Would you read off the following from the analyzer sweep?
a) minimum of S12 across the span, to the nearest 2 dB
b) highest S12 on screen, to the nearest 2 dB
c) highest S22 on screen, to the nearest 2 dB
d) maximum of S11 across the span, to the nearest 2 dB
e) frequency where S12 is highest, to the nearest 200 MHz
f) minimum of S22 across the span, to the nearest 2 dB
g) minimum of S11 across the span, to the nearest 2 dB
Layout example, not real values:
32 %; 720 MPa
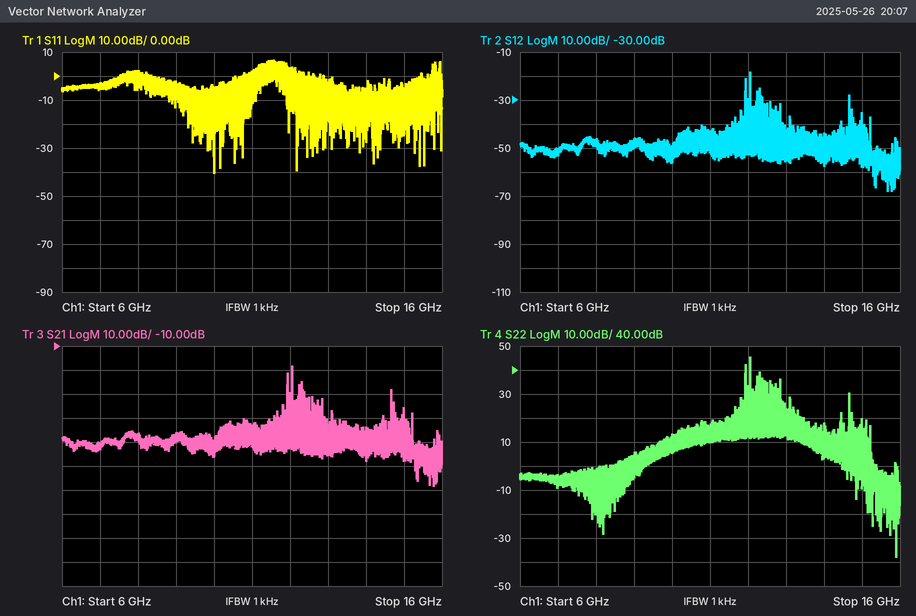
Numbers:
-68 dB; -18 dB; 46 dB; 6 dB; 12.0 GHz; -38 dB; -40 dB
